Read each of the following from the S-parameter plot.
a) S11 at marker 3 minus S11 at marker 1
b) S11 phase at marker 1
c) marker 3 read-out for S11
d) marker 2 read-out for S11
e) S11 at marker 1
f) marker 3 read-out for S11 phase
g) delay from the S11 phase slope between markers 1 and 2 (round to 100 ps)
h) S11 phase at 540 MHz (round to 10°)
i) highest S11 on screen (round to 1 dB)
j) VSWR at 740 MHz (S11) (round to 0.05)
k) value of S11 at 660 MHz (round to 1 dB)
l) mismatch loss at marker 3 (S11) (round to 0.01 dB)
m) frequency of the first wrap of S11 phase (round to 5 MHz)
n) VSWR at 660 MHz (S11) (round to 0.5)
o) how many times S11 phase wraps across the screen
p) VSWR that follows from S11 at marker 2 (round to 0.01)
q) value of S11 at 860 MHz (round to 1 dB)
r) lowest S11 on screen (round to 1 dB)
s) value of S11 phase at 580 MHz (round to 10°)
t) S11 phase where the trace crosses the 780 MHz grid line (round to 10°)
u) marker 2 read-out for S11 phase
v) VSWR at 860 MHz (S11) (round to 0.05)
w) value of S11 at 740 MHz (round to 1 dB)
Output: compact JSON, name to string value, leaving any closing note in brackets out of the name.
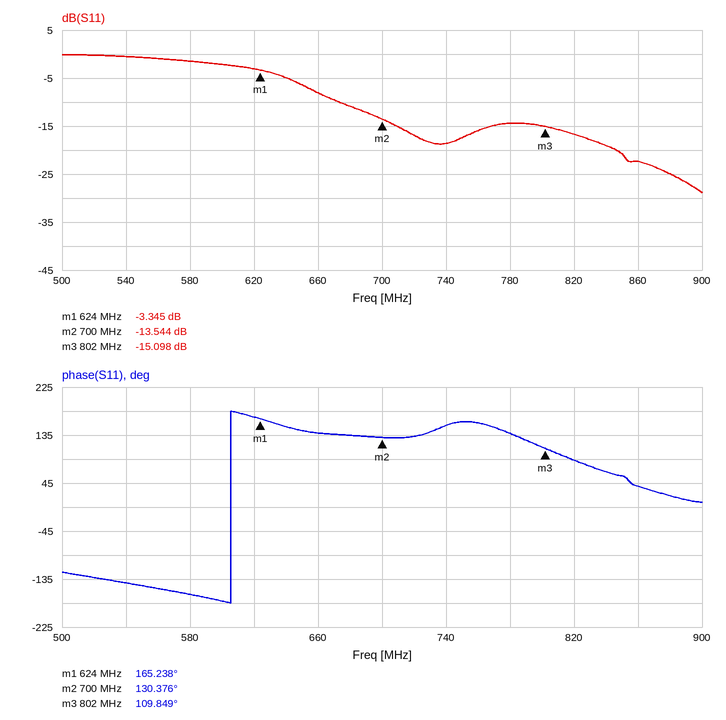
{"S11 at marker 3 minus S11 at marker 1": "-11.753 dB", "S11 phase at marker 1": "165.238°", "marker 3 read-out for S11": "-15.098 dB", "marker 2 read-out for S11": "-13.544 dB", "S11 at marker 1": "-3.345 dB", "marker 3 read-out for S11 phase": "109.849°", "delay from the S11 phase slope between markers 1 and 2": "1.3 ns", "S11 phase at 540 MHz": "-140°", "highest S11 on screen": "0 dB", "VSWR at 740 MHz (S11)": "1.25", "value of S11 at 660 MHz": "-8 dB", "mismatch loss at marker 3 (S11)": "0.14 dB", "frequency of the first wrap of S11 phase": "605 MHz", "VSWR at 660 MHz (S11)": "2.5", "how many times S11 phase wraps across the screen": "1", "VSWR that follows from S11 at marker 2": "1.53", "value of S11 at 860 MHz": "-22 dB", "lowest S11 on screen": "-29 dB", "value of S11 phase at 580 MHz": "-160°", "S11 phase where the trace crosses the 780 MHz grid line": "140°", "marker 2 read-out for S11 phase": "130.376°", "VSWR at 860 MHz (S11)": "1.15", "value of S11 at 740 MHz": "-19 dB"}
